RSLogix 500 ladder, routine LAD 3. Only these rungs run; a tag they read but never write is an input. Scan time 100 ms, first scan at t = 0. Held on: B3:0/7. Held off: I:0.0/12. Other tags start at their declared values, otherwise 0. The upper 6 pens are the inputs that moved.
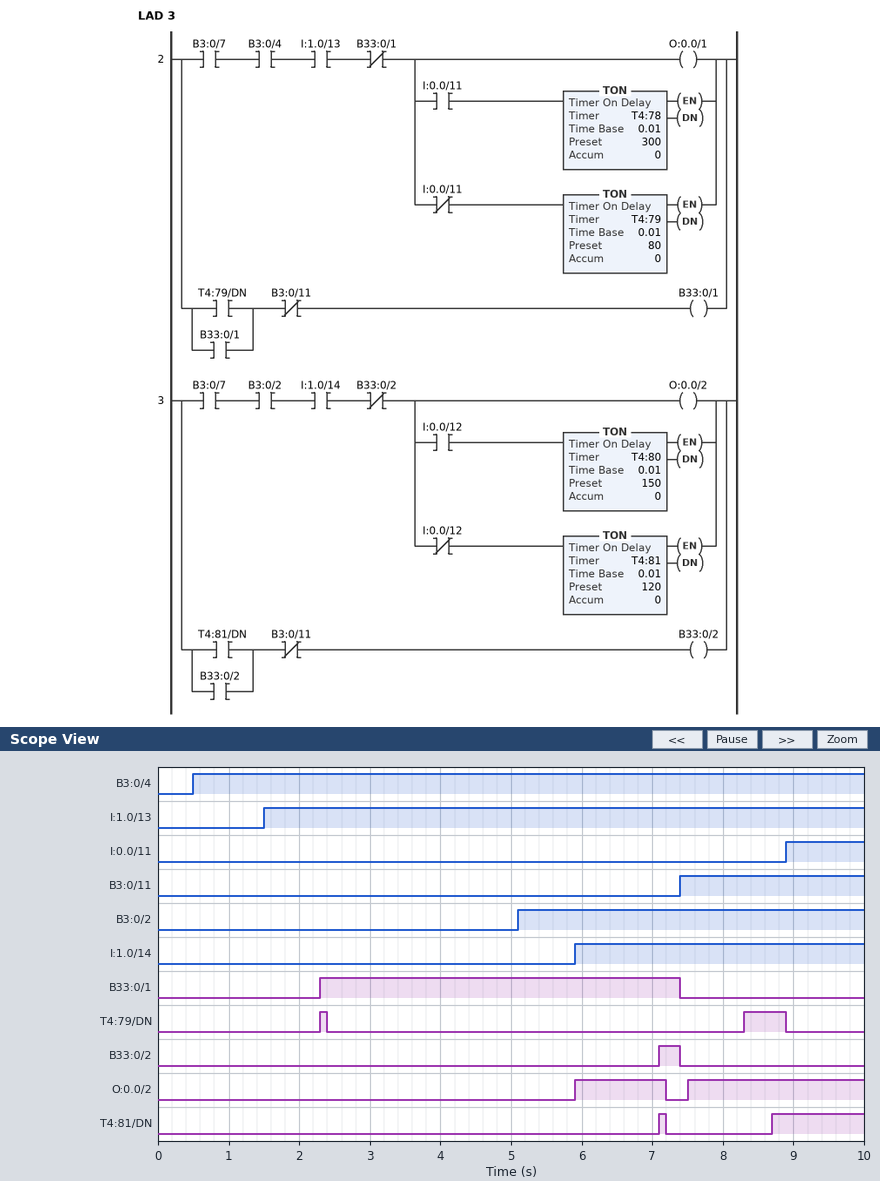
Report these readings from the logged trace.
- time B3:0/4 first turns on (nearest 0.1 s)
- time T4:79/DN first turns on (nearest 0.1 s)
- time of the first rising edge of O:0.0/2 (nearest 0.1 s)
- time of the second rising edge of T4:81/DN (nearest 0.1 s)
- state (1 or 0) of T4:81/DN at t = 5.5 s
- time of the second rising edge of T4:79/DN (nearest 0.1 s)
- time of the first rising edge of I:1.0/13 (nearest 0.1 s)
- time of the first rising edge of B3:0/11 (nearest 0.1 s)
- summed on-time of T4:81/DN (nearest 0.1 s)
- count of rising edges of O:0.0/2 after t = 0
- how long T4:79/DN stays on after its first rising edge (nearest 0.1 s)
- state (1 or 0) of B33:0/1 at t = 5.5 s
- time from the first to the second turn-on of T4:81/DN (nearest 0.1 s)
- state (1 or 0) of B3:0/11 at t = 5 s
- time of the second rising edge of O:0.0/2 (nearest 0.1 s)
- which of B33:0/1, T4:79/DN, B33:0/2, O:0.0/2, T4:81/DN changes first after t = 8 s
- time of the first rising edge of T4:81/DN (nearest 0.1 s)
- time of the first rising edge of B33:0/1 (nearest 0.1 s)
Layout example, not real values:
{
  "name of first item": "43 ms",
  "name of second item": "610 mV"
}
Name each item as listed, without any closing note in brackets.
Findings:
{
  "time B3:0/4 first turns on": "0.5 s",
  "time T4:79/DN first turns on": "2.3 s",
  "time of the first rising edge of O:0.0/2": "5.9 s",
  "time of the second rising edge of T4:81/DN": "8.7 s",
  "state (1 or 0) of T4:81/DN at t = 5.5 s": "0",
  "time of the second rising edge of T4:79/DN": "8.3 s",
  "time of the first rising edge of I:1.0/13": "1.5 s",
  "time of the first rising edge of B3:0/11": "7.4 s",
  "summed on-time of T4:81/DN": "1.4 s",
  "count of rising edges of O:0.0/2 after t = 0": "2",
  "how long T4:79/DN stays on after its first rising edge": "0.1 s",
  "state (1 or 0) of B33:0/1 at t = 5.5 s": "1",
  "time from the first to the second turn-on of T4:81/DN": "1.6 s",
  "state (1 or 0) of B3:0/11 at t = 5 s": "0",
  "time of the second rising edge of O:0.0/2": "7.5 s",
  "which of B33:0/1, T4:79/DN, B33:0/2, O:0.0/2, T4:81/DN changes first after t = 8 s": "T4:79/DN",
  "time of the first rising edge of T4:81/DN": "7.1 s",
  "time of the first rising edge of B33:0/1": "2.3 s"
}
